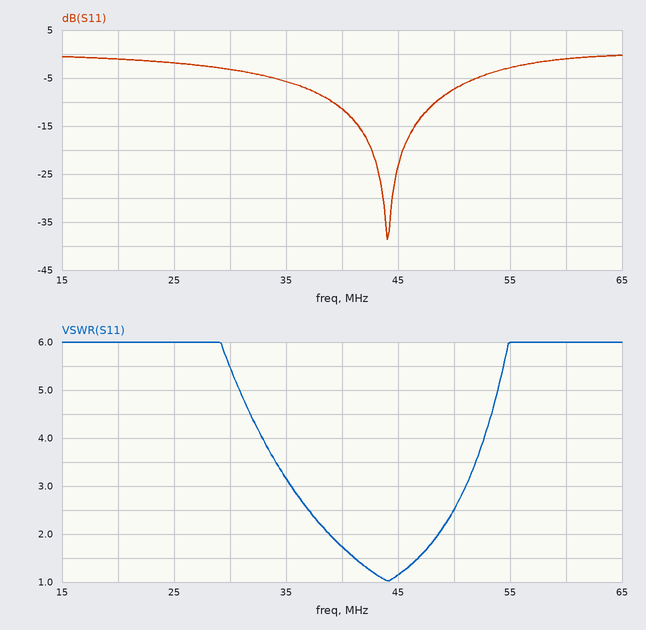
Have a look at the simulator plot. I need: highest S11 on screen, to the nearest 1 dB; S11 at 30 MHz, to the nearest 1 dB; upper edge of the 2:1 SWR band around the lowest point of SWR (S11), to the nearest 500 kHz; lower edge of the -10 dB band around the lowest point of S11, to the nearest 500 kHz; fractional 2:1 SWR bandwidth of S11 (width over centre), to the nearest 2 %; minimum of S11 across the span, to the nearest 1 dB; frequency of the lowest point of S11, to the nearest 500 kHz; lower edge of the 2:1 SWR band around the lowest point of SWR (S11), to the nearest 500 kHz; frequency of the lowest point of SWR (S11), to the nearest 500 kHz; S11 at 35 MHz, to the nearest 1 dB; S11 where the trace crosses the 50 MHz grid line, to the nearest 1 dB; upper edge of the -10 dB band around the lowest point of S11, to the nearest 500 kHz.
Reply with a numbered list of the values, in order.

1. 0 dB
2. -3 dB
3. 48.5 MHz
4. 39.0 MHz
5. 22 %
6. -39 dB
7. 44.0 MHz
8. 39.0 MHz
9. 44.0 MHz
10. -6 dB
11. -7 dB
12. 48.5 MHz
